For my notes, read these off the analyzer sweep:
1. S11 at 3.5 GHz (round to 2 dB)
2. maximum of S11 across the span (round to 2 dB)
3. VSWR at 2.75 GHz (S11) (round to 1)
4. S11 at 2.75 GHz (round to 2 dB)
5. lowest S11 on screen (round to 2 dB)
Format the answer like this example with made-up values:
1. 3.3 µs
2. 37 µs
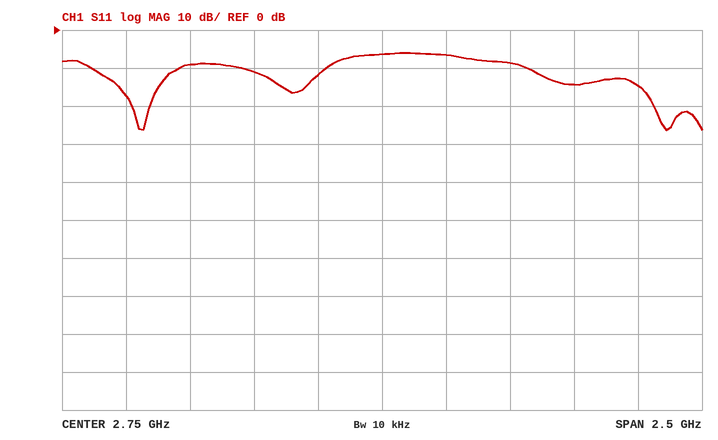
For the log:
1. -14 dB
2. -6 dB
3. 3
4. -6 dB
5. -26 dB
